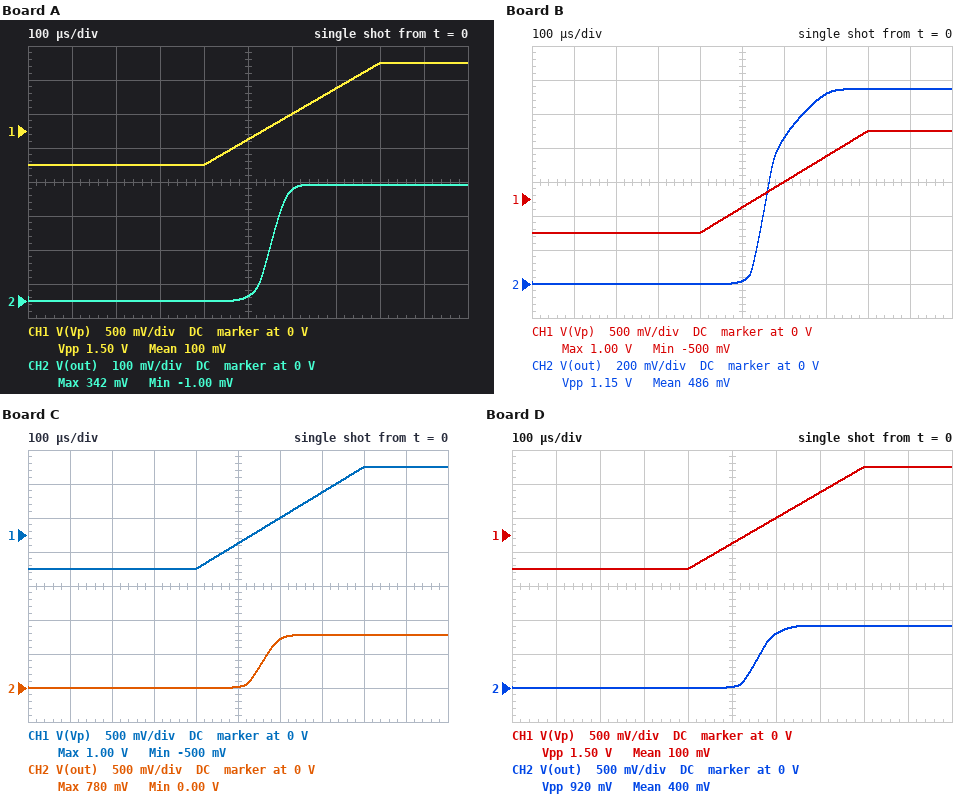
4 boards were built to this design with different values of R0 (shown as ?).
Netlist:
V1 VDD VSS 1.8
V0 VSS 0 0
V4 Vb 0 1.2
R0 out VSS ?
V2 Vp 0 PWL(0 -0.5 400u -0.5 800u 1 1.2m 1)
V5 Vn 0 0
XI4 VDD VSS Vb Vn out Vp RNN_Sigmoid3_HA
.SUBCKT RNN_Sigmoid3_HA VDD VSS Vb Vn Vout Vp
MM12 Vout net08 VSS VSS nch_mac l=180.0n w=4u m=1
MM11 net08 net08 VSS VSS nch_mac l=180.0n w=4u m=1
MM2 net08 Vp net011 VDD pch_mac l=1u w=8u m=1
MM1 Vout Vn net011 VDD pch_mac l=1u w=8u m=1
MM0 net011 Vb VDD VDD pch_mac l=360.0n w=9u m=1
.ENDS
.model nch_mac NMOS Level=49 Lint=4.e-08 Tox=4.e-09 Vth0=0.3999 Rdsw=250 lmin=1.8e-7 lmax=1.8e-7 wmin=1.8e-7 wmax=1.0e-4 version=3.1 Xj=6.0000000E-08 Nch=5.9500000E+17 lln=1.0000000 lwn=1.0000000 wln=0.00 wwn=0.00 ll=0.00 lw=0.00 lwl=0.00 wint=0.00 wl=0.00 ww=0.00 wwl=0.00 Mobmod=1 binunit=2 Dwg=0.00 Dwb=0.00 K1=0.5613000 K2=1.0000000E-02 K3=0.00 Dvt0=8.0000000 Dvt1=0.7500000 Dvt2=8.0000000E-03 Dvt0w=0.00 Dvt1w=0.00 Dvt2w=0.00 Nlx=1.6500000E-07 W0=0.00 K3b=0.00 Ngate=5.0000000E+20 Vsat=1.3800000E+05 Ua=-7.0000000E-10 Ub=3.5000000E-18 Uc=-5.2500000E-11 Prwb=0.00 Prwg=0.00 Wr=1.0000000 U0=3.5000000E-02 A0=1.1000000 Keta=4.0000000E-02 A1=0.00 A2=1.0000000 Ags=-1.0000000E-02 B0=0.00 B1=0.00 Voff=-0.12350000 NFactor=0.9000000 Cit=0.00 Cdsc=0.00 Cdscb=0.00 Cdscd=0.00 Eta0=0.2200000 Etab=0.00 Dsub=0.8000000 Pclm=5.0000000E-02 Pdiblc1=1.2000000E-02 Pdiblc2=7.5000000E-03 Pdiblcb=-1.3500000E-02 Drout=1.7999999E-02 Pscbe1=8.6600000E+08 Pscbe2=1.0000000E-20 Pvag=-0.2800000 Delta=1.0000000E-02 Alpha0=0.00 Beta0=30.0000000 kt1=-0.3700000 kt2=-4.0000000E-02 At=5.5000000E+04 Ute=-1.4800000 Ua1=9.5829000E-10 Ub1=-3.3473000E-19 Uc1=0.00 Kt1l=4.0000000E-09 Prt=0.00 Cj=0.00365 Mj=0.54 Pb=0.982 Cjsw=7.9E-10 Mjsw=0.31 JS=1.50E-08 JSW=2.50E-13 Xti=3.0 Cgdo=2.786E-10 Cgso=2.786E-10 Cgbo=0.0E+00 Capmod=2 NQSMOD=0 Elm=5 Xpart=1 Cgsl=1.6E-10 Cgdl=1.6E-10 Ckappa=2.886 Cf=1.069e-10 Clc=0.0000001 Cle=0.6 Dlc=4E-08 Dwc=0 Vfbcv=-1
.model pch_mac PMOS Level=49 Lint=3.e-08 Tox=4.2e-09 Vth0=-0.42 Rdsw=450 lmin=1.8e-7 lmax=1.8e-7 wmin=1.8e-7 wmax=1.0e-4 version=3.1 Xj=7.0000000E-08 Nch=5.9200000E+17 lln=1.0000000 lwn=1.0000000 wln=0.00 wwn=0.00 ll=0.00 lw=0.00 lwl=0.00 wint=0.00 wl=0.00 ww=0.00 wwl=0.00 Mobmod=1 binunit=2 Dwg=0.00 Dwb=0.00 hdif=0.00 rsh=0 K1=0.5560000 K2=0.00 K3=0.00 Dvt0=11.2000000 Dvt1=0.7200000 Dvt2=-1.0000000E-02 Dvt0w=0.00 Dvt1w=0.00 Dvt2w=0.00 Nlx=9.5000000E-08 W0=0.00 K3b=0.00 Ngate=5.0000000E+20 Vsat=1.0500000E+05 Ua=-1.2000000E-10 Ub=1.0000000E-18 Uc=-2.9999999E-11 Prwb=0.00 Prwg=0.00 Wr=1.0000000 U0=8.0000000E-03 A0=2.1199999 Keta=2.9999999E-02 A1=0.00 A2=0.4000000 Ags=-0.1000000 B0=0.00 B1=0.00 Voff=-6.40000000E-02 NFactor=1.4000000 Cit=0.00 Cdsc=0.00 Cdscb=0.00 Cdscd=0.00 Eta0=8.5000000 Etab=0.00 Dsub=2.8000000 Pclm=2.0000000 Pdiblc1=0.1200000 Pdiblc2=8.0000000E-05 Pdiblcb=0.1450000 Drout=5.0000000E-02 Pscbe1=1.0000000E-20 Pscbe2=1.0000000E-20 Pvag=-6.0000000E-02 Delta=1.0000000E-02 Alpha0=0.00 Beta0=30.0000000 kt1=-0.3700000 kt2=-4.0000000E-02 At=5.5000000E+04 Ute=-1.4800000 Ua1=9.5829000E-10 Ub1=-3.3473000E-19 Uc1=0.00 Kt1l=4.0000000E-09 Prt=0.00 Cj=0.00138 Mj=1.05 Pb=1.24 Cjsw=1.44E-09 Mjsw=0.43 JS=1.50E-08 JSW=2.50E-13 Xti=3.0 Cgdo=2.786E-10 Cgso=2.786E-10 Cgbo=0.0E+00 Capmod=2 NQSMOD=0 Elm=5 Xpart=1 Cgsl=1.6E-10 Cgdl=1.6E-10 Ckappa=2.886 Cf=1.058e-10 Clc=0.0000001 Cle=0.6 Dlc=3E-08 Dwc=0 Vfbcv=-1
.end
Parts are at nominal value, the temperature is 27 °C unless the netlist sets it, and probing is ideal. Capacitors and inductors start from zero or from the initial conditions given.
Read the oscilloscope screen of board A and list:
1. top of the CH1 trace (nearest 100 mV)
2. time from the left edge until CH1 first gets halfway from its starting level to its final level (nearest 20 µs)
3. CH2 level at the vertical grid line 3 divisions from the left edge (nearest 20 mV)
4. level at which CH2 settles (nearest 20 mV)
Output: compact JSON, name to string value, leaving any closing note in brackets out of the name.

{"top of the CH1 trace": "1.0 V", "time from the left edge until CH1 first gets halfway from its starting level to its final level": "600 µs", "CH2 level at the vertical grid line 3 divisions from the left edge": "0 V", "level at which CH2 settles": "340 mV"}
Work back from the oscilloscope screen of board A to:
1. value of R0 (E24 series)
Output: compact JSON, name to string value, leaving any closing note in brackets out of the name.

{"value of R0": "27 kΩ"}
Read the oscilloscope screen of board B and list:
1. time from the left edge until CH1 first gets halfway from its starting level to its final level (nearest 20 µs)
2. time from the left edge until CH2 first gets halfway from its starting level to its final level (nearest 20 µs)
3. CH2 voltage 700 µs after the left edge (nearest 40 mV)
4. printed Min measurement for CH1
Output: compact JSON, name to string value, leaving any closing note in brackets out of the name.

{"time from the left edge until CH1 first gets halfway from its starting level to its final level": "600 µs", "time from the left edge until CH2 first gets halfway from its starting level to its final level": "560 µs", "CH2 voltage 700 µs after the left edge": "1.12 V", "printed Min measurement for CH1": "-500 mV"}
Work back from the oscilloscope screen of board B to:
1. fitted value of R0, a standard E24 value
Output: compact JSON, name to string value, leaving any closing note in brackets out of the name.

{"fitted value of R0, a standard E24 value": "100 kΩ"}
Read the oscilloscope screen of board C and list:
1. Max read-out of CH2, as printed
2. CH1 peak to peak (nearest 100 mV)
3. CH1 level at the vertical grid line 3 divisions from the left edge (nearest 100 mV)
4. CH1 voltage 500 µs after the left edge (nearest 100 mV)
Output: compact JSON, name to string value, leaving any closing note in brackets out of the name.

{"Max read-out of CH2, as printed": "780 mV", "CH1 peak to peak": "1.5 V", "CH1 level at the vertical grid line 3 divisions from the left edge": "-500 mV", "CH1 voltage 500 µs after the left edge": "-100 mV"}
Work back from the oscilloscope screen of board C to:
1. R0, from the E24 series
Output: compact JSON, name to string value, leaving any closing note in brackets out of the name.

{"R0, from the E24 series": "62 kΩ"}
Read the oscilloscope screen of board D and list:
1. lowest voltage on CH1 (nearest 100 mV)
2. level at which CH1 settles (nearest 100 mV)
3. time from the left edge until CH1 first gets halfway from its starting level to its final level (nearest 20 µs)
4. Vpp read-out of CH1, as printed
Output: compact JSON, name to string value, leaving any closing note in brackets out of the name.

{"lowest voltage on CH1": "-500 mV", "level at which CH1 settles": "1.0 V", "time from the left edge until CH1 first gets halfway from its starting level to its final level": "600 µs", "Vpp read-out of CH1, as printed": "1.50 V"}
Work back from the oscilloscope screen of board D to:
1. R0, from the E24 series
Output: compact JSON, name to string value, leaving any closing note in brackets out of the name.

{"R0, from the E24 series": "75 kΩ"}
